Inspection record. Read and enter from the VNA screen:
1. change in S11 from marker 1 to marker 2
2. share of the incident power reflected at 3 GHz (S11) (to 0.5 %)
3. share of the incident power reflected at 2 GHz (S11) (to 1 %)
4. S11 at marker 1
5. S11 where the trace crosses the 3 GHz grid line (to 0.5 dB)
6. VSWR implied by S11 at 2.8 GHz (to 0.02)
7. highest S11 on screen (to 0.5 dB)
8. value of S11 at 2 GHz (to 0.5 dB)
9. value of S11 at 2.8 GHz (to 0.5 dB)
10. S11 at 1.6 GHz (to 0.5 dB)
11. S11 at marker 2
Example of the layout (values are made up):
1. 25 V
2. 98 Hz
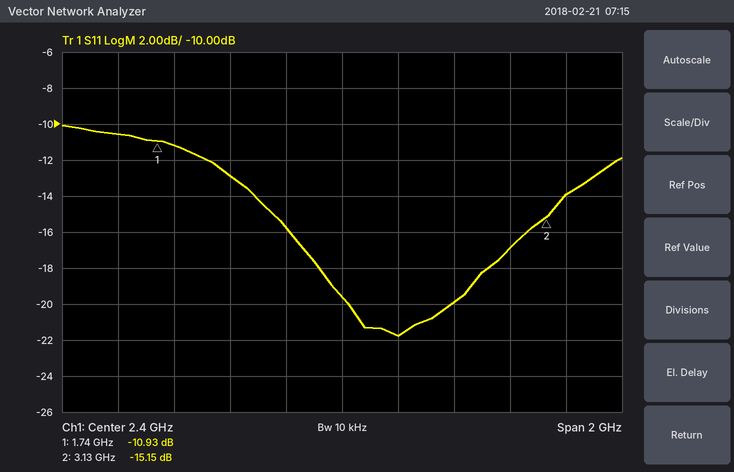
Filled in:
1. -4.22 dB
2. 2.0 %
3. 5 %
4. -10.93 dB
5. -17.0 dB
6. 1.22
7. -10.0 dB
8. -13.0 dB
9. -20.0 dB
10. -10.5 dB
11. -15.15 dB
